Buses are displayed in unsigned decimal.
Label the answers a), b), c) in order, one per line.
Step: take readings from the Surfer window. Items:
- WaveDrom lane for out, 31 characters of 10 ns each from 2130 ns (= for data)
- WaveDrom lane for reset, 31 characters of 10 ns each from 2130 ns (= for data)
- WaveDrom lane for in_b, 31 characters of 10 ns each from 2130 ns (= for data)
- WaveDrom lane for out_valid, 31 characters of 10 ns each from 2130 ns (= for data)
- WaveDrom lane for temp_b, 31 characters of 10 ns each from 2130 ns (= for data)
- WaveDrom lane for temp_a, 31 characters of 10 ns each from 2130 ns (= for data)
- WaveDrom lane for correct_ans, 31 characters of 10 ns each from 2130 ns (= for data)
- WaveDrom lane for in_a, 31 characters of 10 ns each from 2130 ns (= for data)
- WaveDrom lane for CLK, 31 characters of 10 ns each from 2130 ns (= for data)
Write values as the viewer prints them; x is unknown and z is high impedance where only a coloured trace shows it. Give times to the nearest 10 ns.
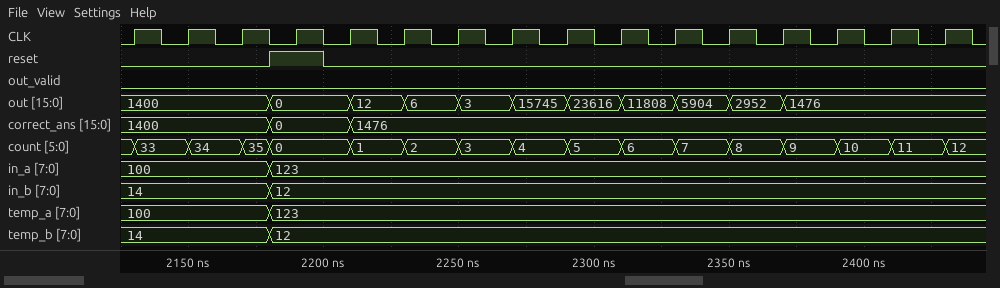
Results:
a) {name: 'out', wave: '=....=..=.=.=.=.=.=.=.=.=......', data: '1400 0 12 6 3 15745 23616 11808 5904 2952 1476'}
b) {name: 'reset', wave: '0....1.0.......................'}
c) {name: 'in_b', wave: '=....=.........................', data: '14 12'}
d) {name: 'out_valid', wave: '0..............................'}
e) {name: 'temp_b', wave: '=....=.........................', data: '14 12'}
f) {name: 'temp_a', wave: '=....=.........................', data: '100 123'}
g) {name: 'correct_ans', wave: '=....=..=......................', data: '1400 0 1476'}
h) {name: 'in_a', wave: '=....=.........................', data: '100 123'}
i) {name: 'CLK', wave: '1010101010101010101010101010101'}
